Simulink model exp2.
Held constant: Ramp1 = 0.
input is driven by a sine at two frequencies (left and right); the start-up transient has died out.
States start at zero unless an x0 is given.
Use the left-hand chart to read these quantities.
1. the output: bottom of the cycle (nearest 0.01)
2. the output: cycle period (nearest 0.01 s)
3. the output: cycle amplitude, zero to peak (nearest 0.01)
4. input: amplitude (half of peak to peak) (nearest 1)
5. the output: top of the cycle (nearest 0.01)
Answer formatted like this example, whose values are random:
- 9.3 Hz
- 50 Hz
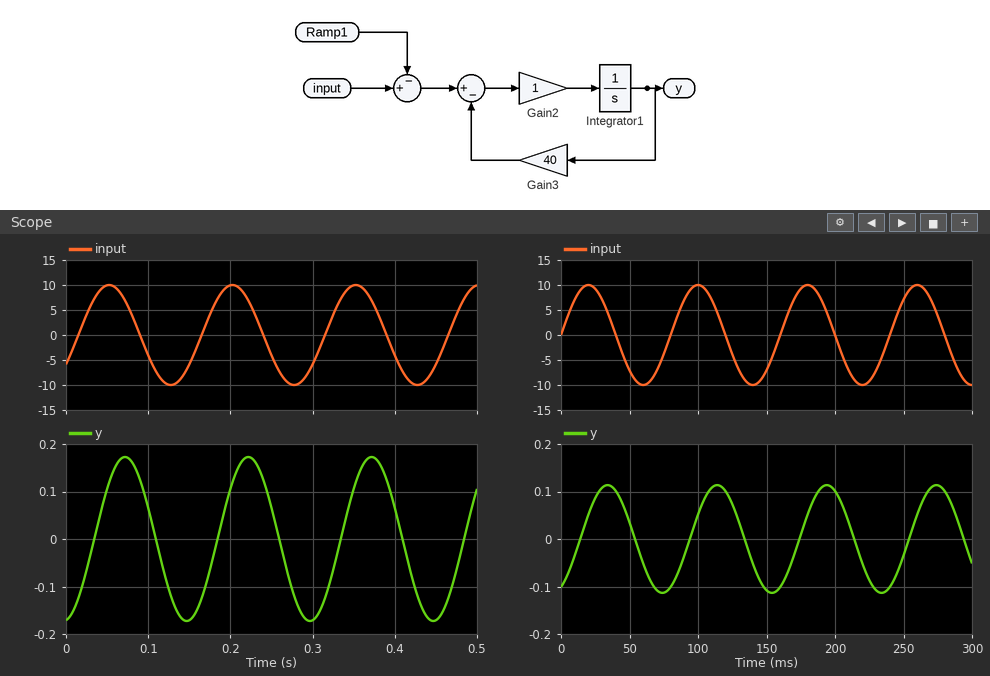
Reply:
- -0.17
- 0.15 s
- 0.17
- 10
- 0.17
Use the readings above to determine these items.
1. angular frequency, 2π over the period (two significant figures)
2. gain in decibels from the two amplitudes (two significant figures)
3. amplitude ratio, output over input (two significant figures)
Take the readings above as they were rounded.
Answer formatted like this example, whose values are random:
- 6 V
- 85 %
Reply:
- 42 rad/s
- -35 dB
- 0.017
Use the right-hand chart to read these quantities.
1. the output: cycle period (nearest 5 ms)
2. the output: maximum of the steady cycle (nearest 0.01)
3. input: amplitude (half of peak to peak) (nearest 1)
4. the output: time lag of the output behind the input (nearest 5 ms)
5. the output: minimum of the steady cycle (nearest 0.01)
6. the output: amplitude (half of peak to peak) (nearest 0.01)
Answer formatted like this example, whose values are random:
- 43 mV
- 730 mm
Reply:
- 80 ms
- 0.11
- 10
- 15 ms
- -0.11
- 0.11
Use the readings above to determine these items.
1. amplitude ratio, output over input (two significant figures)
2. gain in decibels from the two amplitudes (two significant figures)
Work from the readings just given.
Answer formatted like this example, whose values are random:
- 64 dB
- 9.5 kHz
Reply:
- 0.011
- -39 dB
